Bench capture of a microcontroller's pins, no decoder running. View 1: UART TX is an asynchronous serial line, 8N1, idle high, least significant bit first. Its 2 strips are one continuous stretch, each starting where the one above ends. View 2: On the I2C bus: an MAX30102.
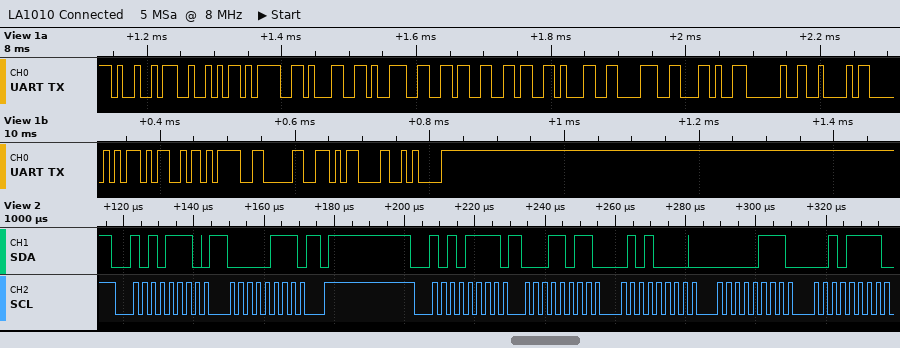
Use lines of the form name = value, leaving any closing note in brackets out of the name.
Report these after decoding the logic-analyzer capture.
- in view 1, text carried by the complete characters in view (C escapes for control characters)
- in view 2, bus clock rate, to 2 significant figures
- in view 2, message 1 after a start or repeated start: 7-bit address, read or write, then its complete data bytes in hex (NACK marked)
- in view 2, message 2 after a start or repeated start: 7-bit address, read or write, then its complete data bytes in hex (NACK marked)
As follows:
in view 1, text carried by the complete characters in view = "IR=196618, BPM=0\r\n"
in view 2, bus clock rate, to 2 significant figures = 400 kHz
in view 2, message 1 after a start or repeated start: 7-bit address, read or write, then its complete data bytes in hex = 0x57 write: 07
in view 2, message 2 after a start or repeated start: 7-bit address, read or write, then its complete data bytes in hex = 0x57 read: 1B 50 07 2F
